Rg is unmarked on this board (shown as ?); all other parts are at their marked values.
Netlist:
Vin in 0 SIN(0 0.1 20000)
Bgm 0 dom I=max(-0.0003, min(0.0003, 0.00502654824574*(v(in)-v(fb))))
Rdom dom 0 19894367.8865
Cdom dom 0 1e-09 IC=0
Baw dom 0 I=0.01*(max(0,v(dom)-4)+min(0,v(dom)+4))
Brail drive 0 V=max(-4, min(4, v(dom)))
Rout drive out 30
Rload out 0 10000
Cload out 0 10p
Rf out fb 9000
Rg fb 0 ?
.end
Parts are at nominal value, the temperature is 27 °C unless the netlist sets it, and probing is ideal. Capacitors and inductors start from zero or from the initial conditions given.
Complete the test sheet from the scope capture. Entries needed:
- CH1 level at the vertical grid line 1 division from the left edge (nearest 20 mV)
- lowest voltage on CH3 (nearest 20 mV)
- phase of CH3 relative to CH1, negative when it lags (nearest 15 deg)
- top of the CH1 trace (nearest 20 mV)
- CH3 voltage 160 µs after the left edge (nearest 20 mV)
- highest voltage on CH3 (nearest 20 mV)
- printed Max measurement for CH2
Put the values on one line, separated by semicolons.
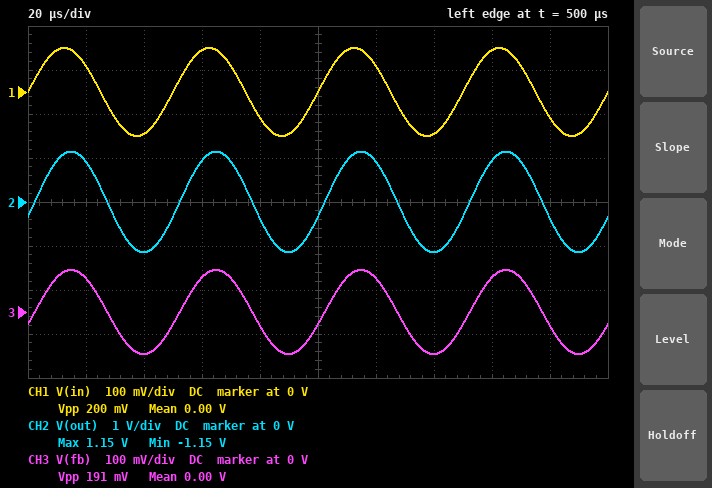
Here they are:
60 mV; -100 mV; -15 deg; 100 mV; 80 mV; 100 mV; 1.15 V
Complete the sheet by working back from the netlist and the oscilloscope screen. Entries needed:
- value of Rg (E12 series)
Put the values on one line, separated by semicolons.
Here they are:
820 Ω
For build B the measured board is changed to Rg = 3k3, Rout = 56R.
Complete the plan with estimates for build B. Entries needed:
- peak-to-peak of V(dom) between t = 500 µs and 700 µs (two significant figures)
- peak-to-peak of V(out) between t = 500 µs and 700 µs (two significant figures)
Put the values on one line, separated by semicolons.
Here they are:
750 mV; 740 mV
